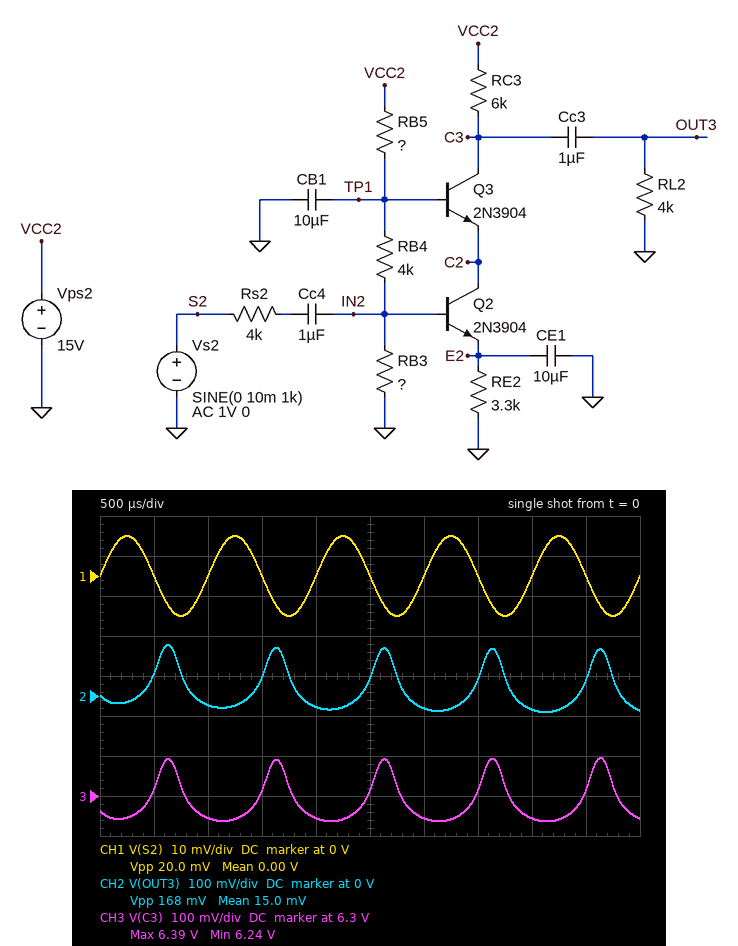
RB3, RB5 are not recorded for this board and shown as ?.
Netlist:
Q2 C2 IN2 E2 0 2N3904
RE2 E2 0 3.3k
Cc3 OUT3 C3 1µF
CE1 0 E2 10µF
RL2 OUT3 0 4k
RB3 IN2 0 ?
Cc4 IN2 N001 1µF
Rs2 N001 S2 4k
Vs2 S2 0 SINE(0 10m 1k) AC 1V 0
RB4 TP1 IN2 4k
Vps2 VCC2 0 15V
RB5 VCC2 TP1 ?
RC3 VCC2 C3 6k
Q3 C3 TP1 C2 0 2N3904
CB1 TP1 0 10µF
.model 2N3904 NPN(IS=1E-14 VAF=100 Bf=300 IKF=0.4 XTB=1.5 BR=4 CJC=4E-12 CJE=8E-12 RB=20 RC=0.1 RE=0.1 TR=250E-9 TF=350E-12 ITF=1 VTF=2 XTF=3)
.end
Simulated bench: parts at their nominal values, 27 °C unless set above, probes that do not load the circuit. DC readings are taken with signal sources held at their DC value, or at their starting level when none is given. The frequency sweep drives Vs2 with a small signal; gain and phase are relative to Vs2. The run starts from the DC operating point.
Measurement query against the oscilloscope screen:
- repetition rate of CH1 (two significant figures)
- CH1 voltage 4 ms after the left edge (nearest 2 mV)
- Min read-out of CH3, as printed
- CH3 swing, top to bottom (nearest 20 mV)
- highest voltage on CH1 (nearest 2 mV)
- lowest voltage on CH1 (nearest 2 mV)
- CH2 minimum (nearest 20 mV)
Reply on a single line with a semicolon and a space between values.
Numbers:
1.0 kHz; 0 V; 6.24 V; 160 mV; 10 mV; -10 mV; -40 mV
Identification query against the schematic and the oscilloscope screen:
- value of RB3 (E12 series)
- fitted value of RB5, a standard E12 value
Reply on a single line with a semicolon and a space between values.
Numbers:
22 kΩ; 22 kΩ
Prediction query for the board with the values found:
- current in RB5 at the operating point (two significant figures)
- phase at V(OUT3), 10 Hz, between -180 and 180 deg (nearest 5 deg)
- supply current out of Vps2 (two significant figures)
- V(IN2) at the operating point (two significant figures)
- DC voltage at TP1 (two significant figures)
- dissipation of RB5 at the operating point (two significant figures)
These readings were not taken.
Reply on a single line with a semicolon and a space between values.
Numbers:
370 µA; -10 deg; 1.8 mA; 5.8 V; 6.9 V; 3.0 mW
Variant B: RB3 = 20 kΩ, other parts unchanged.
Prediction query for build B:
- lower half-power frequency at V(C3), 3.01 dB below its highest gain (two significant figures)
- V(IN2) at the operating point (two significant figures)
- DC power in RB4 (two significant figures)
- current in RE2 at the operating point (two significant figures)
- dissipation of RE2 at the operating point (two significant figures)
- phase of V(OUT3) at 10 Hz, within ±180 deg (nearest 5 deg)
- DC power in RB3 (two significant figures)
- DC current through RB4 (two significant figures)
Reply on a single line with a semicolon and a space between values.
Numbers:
950 Hz; 5.7 V; 340 µW; 1.5 mA; 7.8 mW; -10 deg; 1.6 mW; 290 µA
